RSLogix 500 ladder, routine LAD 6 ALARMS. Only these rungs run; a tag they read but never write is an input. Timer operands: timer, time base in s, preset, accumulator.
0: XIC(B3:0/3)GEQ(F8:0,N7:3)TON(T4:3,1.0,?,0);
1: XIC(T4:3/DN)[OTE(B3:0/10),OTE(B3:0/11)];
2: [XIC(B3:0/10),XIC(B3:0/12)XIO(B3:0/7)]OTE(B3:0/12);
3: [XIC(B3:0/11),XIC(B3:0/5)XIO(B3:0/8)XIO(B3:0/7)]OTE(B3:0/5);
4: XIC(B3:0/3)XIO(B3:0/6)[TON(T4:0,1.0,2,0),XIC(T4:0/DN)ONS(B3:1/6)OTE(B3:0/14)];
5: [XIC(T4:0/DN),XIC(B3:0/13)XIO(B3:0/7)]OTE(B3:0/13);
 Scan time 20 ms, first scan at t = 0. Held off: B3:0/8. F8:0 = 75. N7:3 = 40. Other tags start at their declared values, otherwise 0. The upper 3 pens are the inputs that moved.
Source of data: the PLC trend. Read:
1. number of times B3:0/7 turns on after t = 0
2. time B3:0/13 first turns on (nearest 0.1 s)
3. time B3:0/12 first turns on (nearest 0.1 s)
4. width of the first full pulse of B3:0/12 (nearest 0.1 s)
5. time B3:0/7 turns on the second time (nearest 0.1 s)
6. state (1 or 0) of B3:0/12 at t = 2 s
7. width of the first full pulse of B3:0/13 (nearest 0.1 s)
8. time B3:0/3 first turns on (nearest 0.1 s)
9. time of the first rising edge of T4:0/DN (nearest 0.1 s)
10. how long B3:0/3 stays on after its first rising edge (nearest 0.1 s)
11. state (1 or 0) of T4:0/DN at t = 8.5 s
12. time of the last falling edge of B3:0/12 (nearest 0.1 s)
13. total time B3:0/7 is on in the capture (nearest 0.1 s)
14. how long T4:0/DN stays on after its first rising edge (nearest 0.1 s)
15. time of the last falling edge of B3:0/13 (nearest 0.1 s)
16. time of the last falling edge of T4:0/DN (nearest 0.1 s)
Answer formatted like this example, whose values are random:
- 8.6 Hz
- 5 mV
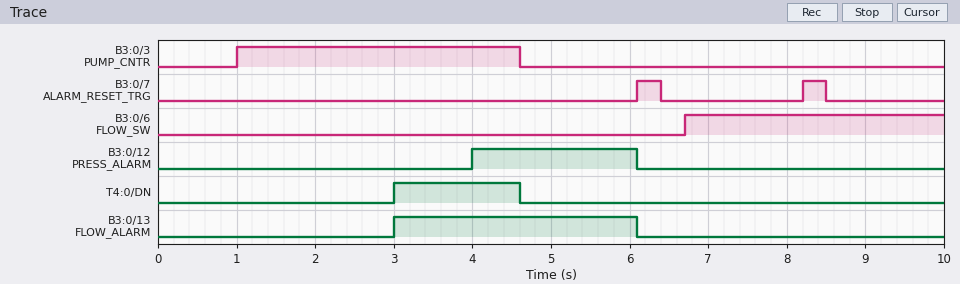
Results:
- 2
- 3.0 s
- 4.0 s
- 2.1 s
- 8.2 s
- 0
- 3.1 s
- 1.0 s
- 3.0 s
- 3.6 s
- 0
- 6.1 s
- 0.6 s
- 1.6 s
- 6.1 s
- 4.6 s
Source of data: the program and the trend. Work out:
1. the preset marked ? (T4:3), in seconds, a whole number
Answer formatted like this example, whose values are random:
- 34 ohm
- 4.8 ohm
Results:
- 3 s
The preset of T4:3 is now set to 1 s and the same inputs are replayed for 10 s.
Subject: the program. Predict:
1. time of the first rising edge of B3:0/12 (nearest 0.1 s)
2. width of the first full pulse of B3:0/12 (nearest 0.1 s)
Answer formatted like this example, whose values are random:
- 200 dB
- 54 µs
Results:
- 2.0 s
- 4.1 s
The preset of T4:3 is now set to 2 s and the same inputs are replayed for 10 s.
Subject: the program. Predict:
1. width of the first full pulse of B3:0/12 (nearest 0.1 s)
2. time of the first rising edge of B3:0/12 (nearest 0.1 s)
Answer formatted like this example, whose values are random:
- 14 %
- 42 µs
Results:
- 3.1 s
- 3.0 s
